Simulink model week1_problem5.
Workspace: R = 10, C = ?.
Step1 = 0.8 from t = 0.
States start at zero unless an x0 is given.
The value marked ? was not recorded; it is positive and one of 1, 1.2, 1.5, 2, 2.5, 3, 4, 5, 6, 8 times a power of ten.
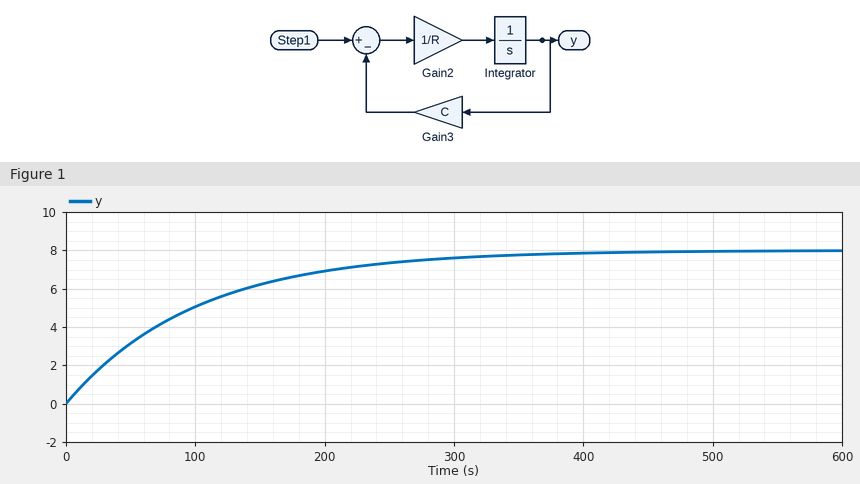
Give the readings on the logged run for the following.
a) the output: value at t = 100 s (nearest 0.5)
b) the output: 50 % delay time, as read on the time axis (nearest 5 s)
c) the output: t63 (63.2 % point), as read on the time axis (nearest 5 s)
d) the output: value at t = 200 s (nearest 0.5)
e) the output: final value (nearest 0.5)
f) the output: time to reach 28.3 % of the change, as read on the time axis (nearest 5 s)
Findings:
5.0
70 s
100 s
7.0
8.0
35 s
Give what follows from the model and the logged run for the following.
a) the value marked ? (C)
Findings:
0.1
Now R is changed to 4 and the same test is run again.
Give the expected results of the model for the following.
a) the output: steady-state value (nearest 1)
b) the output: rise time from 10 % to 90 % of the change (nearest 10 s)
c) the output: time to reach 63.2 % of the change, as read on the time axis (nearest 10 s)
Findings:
8
90 s
40 s
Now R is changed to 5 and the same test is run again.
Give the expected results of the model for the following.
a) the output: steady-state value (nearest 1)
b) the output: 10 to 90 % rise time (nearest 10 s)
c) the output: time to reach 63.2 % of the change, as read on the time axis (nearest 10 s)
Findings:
8
110 s
50 s
